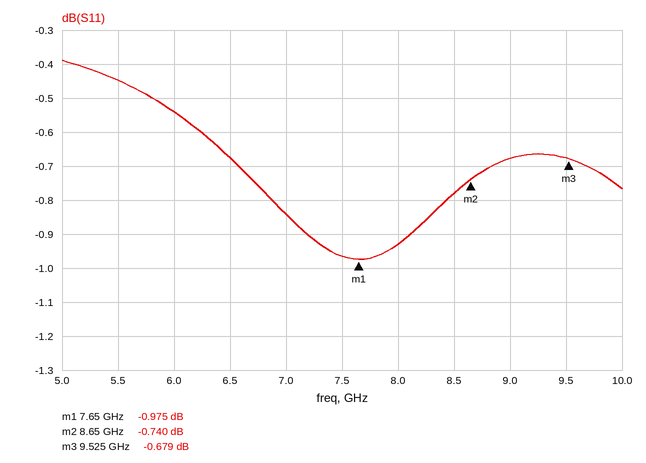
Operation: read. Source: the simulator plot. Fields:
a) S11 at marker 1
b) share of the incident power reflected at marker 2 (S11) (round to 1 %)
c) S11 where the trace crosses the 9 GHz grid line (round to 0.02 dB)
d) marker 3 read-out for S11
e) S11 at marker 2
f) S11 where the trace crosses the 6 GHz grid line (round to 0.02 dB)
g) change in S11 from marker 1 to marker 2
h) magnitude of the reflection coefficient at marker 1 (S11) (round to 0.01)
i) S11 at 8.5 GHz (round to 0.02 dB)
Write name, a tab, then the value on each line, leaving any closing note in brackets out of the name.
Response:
S11 at marker 1	-0.975 dB
share of the incident power reflected at marker 2 (S11)	84 %
S11 where the trace crosses the 9 GHz grid line	-0.68 dB
marker 3 read-out for S11	-0.679 dB
S11 at marker 2	-0.740 dB
S11 where the trace crosses the 6 GHz grid line	-0.54 dB
change in S11 from marker 1 to marker 2	0.235 dB
magnitude of the reflection coefficient at marker 1 (S11)	0.89
S11 at 8.5 GHz	-0.78 dB
